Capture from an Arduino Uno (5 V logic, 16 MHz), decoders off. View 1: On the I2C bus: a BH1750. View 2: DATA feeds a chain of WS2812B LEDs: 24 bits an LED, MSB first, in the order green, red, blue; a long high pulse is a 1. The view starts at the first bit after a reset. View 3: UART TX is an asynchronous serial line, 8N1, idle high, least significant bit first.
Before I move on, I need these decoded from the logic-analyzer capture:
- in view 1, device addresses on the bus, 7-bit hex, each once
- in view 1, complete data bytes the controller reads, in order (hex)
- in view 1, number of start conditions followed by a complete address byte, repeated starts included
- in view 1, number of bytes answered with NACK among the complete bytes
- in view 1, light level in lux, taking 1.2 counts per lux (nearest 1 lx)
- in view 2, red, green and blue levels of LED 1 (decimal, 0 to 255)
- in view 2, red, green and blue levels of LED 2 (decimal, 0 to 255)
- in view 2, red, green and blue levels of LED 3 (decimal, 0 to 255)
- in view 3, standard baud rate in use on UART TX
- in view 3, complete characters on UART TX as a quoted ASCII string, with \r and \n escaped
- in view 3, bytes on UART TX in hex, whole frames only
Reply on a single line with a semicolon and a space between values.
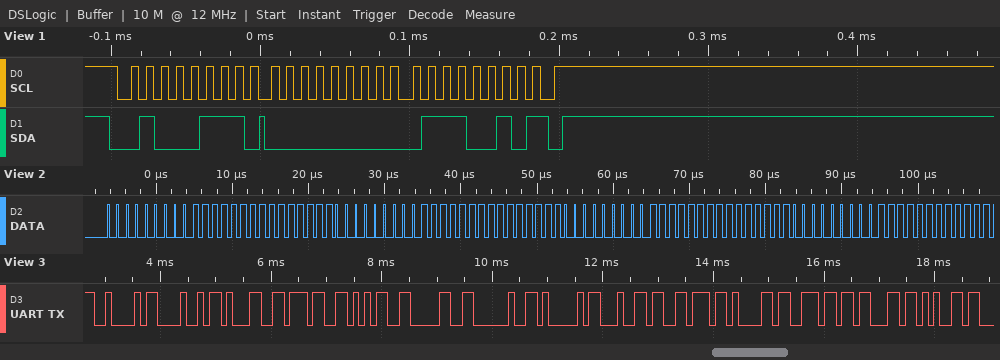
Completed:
0x23; 00 72; 1; 1; 95 lx; 127, 0, 255; 127, 0, 255; 127, 0, 255; 9600 baud; "BH1750 Advance"; 42 48 31 37 35 30 20 41 64 76 61 6E 63 65
